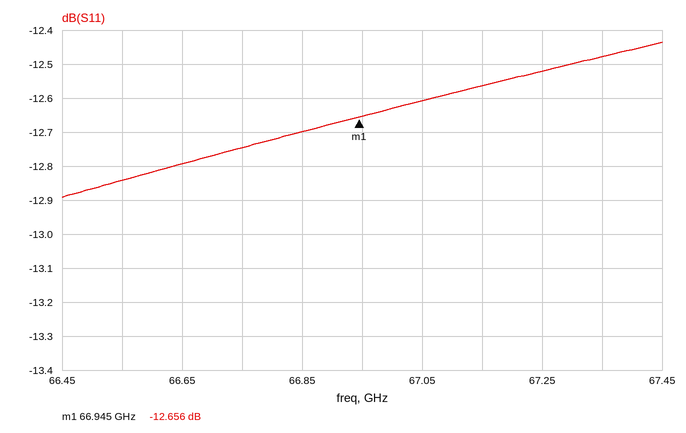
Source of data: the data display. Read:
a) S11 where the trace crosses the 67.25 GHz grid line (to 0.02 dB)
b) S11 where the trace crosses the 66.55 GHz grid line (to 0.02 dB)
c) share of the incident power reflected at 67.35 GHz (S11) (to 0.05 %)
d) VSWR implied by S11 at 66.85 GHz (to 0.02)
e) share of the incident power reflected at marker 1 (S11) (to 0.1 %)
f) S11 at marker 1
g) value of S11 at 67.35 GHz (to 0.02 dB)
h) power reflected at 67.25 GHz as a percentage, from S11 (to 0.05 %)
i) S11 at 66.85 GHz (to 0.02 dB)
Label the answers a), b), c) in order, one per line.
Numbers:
a) -12.52 dB
b) -12.84 dB
c) 5.65 %
d) 1.60
e) 5.4 %
f) -12.656 dB
g) -12.48 dB
h) 5.60 %
i) -12.70 dB
